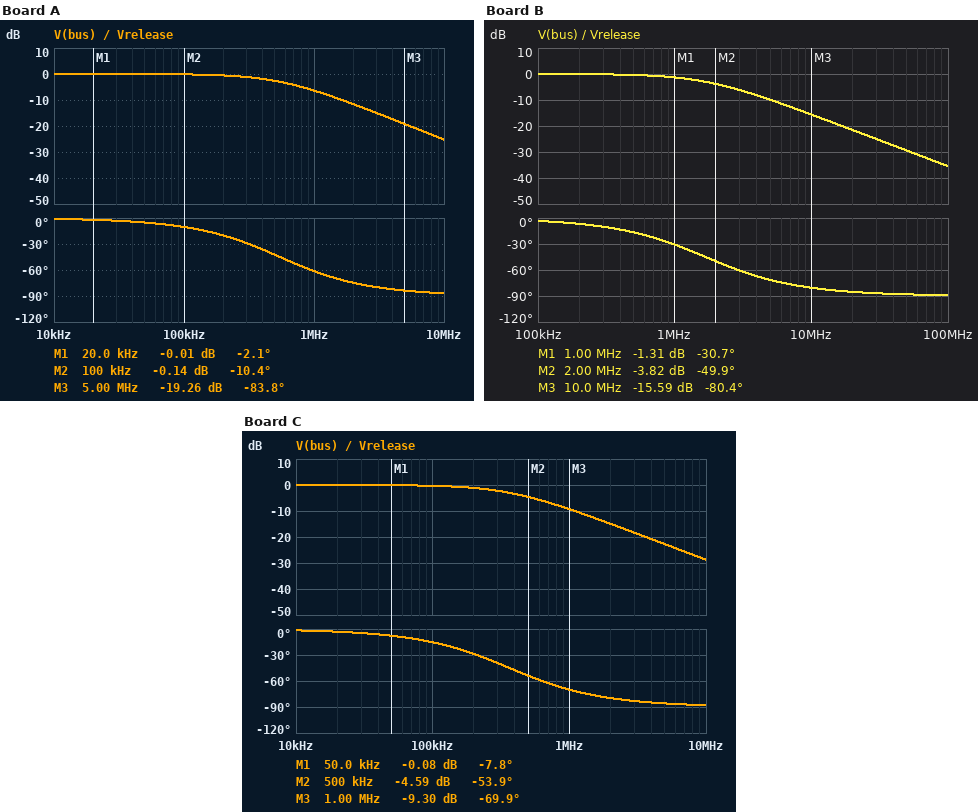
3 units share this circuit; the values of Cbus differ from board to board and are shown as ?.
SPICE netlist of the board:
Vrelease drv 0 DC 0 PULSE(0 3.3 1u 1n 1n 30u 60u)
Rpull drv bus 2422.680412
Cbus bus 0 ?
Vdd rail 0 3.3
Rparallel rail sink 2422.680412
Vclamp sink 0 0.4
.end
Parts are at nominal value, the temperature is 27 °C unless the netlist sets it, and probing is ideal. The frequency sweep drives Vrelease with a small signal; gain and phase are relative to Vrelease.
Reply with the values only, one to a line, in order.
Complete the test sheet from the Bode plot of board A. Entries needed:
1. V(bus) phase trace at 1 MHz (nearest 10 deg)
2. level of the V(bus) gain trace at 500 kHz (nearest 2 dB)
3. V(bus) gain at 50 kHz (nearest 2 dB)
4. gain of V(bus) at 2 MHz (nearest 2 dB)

-60 deg
-2 dB
0 dB
-12 dB
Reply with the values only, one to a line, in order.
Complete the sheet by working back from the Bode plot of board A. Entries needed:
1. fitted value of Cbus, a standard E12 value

120 pF
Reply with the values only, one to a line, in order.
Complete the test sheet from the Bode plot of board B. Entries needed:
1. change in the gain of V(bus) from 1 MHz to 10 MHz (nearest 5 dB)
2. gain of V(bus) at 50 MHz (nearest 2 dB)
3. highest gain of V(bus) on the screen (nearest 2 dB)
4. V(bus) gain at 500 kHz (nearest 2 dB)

-15 dB
-30 dB
0 dB
0 dB
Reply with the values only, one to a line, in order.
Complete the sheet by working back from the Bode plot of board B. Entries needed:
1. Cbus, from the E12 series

39 pF
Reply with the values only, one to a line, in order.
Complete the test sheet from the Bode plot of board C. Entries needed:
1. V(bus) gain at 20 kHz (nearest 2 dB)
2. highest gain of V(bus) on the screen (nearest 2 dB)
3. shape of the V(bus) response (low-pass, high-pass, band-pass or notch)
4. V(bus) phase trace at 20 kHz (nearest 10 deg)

0 dB
0 dB
low-pass
0 deg
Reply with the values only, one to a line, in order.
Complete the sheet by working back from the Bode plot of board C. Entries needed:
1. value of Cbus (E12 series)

180 pF
